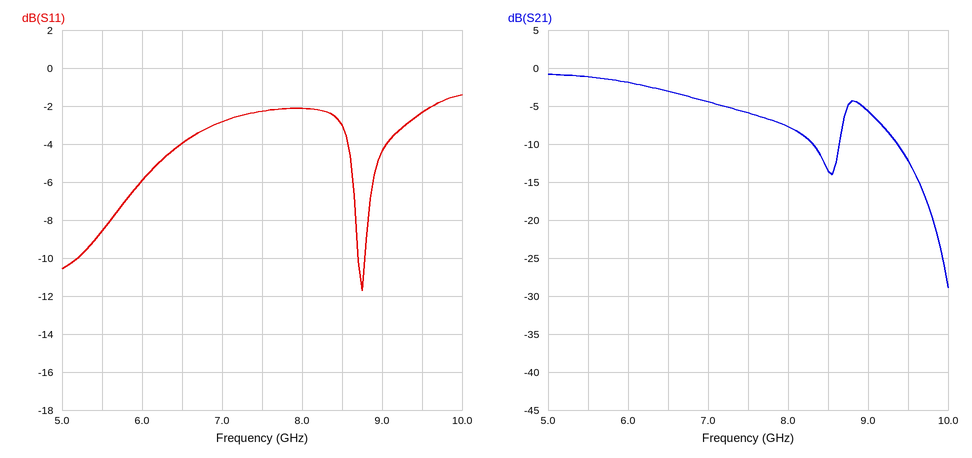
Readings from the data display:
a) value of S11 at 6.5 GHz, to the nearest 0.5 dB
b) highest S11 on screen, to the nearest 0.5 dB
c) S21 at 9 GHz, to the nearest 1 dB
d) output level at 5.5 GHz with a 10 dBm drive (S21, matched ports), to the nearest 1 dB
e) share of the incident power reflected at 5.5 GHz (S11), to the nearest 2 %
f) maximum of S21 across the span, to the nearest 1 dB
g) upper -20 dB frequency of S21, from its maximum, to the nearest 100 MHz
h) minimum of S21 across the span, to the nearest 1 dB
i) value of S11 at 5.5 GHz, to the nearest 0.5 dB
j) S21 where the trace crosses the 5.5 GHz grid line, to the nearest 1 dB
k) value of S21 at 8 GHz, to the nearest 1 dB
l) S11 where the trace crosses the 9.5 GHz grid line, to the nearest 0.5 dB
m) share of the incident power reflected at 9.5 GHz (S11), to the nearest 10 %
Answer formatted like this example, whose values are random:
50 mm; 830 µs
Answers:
-4.0 dB; -1.5 dB; -6 dB; 9 dBm; 14 %; -1 dB; 9.8 GHz; -29 dB; -8.5 dB; -1 dB; -8 dB; -2.5 dB; 60 %
